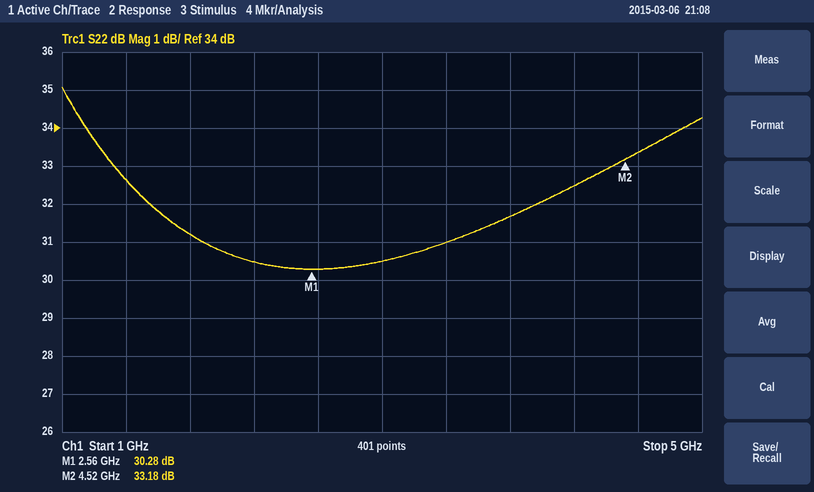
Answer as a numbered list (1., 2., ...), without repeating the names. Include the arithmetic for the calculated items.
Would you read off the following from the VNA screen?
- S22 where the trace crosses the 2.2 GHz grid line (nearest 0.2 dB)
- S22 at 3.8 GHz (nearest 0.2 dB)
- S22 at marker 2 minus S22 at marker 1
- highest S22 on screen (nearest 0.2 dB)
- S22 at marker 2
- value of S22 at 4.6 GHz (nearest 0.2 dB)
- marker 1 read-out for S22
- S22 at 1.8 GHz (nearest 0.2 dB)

1. 30.4 dB
2. 31.6 dB
3. 33.18 − (30.28) = 2.90 dB
4. 35.0 dB
5. 33.18 dB
6. 33.4 dB
7. 30.28 dB
8. 31.2 dB
